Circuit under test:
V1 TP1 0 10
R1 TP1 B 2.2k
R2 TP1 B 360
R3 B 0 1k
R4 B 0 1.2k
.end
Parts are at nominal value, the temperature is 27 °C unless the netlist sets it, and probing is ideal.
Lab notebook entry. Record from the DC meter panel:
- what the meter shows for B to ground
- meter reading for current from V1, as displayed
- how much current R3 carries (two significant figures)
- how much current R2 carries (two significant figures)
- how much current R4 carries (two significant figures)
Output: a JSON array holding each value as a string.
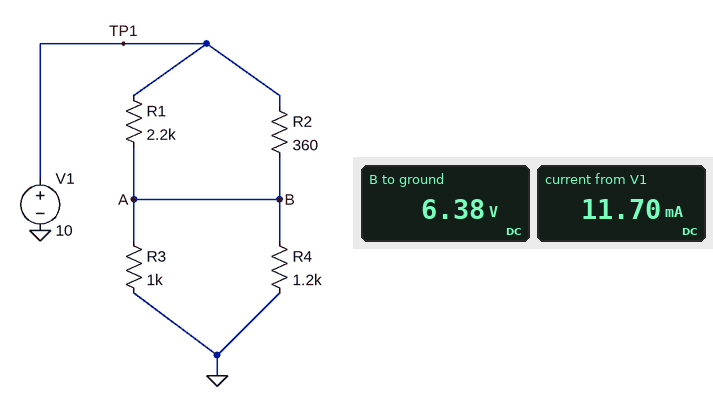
["6.38 V", "11.70 mA", "6.4 mA", "10 mA", "5.3 mA"]
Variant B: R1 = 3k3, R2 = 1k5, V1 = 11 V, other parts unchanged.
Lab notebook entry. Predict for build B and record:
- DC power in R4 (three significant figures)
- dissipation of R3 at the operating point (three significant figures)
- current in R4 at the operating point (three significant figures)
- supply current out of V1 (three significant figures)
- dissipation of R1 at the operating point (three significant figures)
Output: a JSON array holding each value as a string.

["12.1 mW", "14.5 mW", "3.17 mA", "6.98 mA", "15.7 mW"]
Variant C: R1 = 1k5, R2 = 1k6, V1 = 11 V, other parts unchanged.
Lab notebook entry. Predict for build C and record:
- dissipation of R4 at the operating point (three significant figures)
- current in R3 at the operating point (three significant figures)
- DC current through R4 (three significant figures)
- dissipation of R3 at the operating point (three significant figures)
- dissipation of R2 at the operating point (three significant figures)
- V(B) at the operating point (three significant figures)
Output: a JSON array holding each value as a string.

["17.2 mW", "4.55 mA", "3.79 mA", "20.7 mW", "26.0 mW", "4.55 V"]
